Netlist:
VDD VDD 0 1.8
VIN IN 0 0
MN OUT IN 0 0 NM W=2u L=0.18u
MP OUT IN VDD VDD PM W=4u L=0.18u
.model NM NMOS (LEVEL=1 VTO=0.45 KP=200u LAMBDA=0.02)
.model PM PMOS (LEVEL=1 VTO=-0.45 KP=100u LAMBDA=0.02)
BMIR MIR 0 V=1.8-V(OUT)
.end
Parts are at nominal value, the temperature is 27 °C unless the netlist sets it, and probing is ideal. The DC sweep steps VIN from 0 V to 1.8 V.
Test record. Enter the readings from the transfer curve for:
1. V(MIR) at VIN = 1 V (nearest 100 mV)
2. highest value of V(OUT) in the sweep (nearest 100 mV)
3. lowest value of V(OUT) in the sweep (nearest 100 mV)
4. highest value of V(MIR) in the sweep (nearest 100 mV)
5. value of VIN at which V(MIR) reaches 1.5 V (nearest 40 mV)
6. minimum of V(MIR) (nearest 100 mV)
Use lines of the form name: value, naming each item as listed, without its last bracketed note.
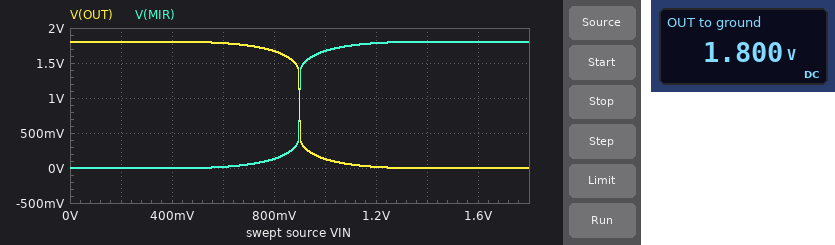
V(MIR) at VIN = 1 V: 1.7 V
highest value of V(OUT) in the sweep: 1.8 V
lowest value of V(OUT) in the sweep: 0 V
highest value of V(MIR) in the sweep: 1.8 V
value of VIN at which V(MIR) reaches 1.5 V: 920 mV
minimum of V(MIR): 0 V
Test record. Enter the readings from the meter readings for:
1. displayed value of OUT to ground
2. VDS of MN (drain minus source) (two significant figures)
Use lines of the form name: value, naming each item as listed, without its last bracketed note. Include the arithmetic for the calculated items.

displayed value of OUT to ground: 1.800 V
VDS of MN (drain minus source): 1.8 V = 1.8 V
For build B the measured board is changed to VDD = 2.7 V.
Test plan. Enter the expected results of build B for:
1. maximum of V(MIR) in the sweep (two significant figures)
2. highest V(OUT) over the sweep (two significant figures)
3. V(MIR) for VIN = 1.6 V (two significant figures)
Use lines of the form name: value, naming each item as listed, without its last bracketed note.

maximum of V(MIR) in the sweep: 1.7 V
highest V(OUT) over the sweep: 2.7 V
V(MIR) for VIN = 1.6 V: 1.6 V
